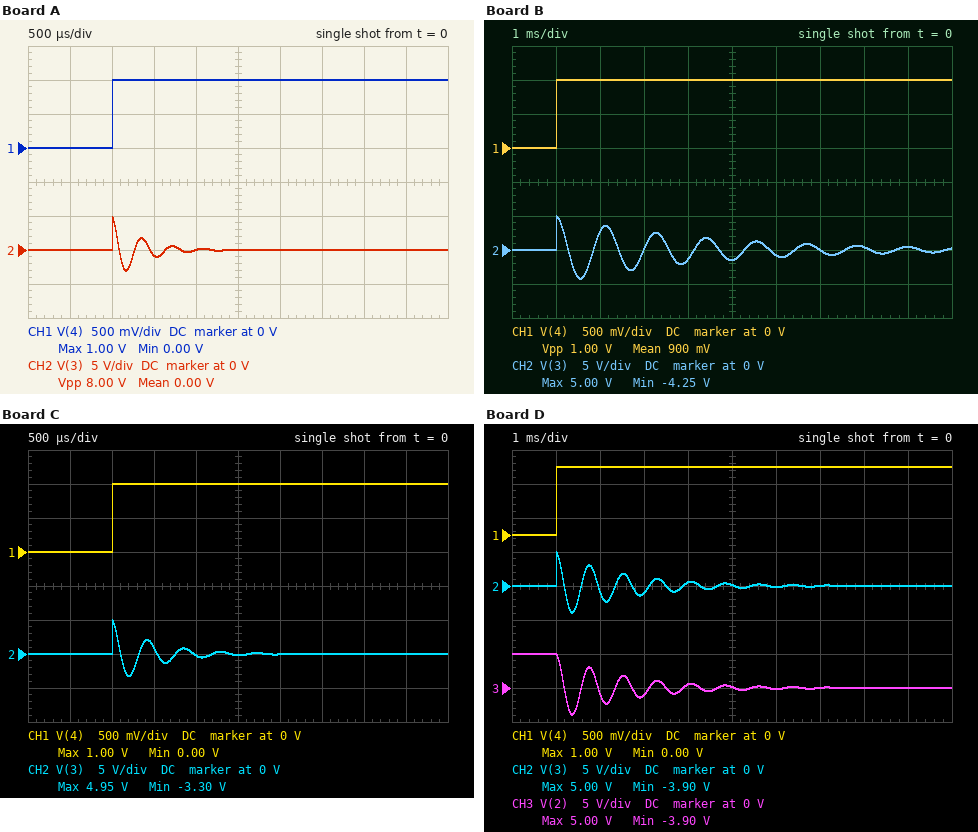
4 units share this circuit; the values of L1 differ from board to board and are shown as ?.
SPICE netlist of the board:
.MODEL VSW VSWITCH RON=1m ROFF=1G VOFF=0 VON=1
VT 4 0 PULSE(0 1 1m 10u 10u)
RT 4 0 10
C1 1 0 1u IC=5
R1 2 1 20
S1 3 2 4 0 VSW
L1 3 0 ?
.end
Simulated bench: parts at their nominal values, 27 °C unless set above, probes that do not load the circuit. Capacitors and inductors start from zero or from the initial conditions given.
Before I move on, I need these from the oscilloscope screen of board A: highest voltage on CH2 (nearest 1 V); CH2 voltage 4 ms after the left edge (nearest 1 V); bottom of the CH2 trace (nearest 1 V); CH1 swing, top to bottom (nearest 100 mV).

5 V
0 V
-3 V
1.0 V
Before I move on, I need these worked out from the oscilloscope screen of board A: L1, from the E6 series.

3.3 mH
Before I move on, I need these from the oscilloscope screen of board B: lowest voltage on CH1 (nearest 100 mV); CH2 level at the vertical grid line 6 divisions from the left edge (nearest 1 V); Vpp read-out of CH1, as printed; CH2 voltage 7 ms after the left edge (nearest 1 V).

0 V
-1 V
1.00 V
0 V
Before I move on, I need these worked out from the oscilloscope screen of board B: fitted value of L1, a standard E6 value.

33 mH
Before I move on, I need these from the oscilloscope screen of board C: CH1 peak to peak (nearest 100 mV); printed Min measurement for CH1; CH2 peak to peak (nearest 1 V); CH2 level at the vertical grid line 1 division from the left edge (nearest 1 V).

1.0 V
0.00 V
8 V
0 V
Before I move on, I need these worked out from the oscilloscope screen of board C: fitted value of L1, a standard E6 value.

4.7 mH
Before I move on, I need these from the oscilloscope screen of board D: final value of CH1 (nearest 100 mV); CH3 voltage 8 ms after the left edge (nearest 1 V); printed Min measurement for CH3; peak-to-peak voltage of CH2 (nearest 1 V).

1.0 V
0 V
-3.90 V
9 V
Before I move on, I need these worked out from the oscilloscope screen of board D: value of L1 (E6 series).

15 mH
